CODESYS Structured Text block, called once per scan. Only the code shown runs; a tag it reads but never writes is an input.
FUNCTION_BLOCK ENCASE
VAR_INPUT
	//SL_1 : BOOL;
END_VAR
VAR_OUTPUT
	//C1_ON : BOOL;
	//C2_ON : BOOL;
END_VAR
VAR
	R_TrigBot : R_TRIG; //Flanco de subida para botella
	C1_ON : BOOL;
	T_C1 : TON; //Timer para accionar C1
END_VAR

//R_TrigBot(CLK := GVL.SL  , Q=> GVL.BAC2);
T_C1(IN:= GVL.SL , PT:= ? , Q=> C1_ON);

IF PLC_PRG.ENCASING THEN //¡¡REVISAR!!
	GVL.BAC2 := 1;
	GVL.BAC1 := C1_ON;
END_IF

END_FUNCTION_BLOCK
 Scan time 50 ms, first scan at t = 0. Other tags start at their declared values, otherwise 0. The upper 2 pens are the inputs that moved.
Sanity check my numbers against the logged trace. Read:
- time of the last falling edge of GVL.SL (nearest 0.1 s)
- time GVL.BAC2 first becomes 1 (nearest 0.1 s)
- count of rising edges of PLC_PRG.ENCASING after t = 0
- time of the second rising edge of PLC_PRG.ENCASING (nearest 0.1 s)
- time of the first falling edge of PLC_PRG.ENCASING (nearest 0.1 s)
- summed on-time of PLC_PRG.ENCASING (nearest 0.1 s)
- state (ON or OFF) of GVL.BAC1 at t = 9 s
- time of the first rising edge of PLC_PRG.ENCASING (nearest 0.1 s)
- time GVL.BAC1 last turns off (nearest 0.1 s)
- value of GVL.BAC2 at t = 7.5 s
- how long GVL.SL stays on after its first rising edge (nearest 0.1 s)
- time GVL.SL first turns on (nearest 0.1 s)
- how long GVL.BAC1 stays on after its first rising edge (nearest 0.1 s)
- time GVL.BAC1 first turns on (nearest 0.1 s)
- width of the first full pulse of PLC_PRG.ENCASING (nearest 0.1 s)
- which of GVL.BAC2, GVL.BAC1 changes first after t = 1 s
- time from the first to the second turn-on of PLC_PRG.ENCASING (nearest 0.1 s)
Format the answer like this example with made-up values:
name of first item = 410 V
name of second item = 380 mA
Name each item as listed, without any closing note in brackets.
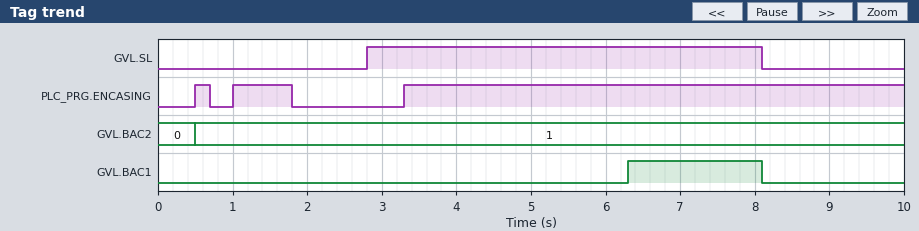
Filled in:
time of the last falling edge of GVL.SL = 8.1 s
time GVL.BAC2 first becomes 1 = 0.5 s
count of rising edges of PLC_PRG.ENCASING after t = 0 = 3
time of the second rising edge of PLC_PRG.ENCASING = 1.0 s
time of the first falling edge of PLC_PRG.ENCASING = 0.7 s
summed on-time of PLC_PRG.ENCASING = 7.7 s
state (ON or OFF) of GVL.BAC1 at t = 9 s = OFF
time of the first rising edge of PLC_PRG.ENCASING = 0.5 s
time GVL.BAC1 last turns off = 8.1 s
value of GVL.BAC2 at t = 7.5 s = 1
how long GVL.SL stays on after its first rising edge = 5.3 s
time GVL.SL first turns on = 2.8 s
how long GVL.BAC1 stays on after its first rising edge = 1.8 s
time GVL.BAC1 first turns on = 6.3 s
width of the first full pulse of PLC_PRG.ENCASING = 0.2 s
which of GVL.BAC2, GVL.BAC1 changes first after t = 1 s = GVL.BAC1
time from the first to the second turn-on of PLC_PRG.ENCASING = 0.5 s
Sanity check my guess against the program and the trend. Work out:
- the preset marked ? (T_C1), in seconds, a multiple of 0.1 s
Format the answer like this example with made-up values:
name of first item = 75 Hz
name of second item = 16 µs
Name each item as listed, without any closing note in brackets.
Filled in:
the preset marked ? (T_C1), in seconds, a multiple of 0.1 s = 3.5 s
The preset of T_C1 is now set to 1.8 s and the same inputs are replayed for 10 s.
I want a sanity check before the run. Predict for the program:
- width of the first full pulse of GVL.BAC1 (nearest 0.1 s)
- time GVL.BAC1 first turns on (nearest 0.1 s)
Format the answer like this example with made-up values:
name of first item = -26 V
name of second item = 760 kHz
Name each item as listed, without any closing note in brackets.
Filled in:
width of the first full pulse of GVL.BAC1 = 3.5 s
time GVL.BAC1 first turns on = 4.6 s
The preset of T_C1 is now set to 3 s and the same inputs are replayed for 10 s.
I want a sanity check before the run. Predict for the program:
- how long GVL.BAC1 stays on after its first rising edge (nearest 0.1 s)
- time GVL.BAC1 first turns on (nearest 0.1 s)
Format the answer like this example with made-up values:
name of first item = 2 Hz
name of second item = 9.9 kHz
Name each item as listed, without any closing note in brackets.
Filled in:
how long GVL.BAC1 stays on after its first rising edge = 2.3 s
time GVL.BAC1 first turns on = 5.8 s
